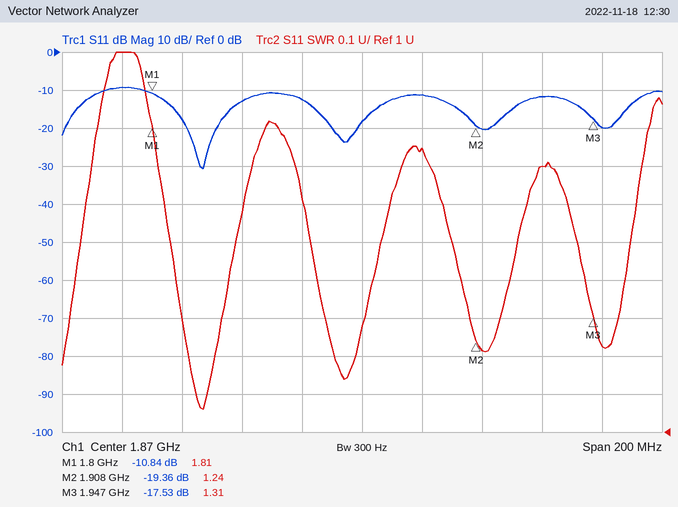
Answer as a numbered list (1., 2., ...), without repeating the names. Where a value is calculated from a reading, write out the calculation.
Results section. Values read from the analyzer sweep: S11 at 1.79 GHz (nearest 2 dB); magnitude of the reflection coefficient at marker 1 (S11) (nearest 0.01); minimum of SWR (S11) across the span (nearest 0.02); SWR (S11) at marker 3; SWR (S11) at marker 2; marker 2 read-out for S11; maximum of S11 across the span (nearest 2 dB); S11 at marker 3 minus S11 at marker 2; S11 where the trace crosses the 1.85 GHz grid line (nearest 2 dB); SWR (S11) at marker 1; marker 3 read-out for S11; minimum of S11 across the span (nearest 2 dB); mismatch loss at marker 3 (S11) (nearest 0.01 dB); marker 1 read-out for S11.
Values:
1. -10 dB
2. 10^(-10.84/20) ≈ 0.29
3. 1.06
4. 1.31
5. 1.24
6. -19.36 dB
7. -10 dB
8. -17.53 − (-19.36) = 1.83 dB
9. -12 dB
10. 1.81
11. -17.53 dB
12. -30 dB
13. −10 log10(1 − 10^(-17.53/10)) ≈ 0.08 dB
14. -10.84 dB
